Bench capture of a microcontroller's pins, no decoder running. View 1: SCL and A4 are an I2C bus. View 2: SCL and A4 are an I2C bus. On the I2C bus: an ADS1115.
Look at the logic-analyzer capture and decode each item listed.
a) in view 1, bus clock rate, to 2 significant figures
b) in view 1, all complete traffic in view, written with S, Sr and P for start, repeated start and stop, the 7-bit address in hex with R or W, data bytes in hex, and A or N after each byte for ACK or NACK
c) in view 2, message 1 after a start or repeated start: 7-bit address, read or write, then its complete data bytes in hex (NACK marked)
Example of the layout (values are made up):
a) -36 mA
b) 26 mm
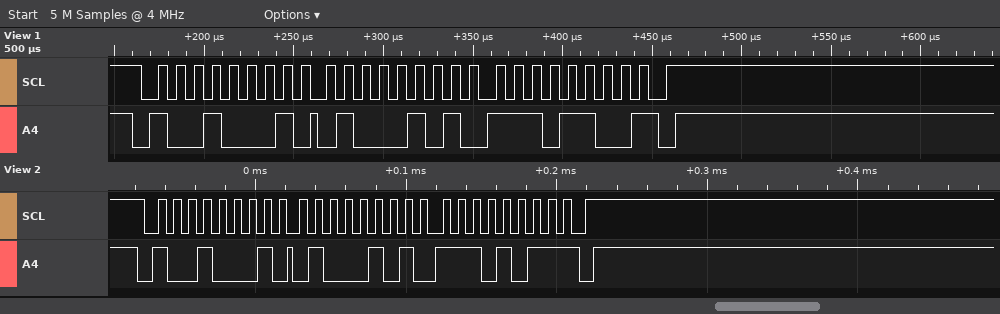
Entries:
a) 100 kHz
b) S 48R A 45 A EC N P
c) 0x48 read: 45 EB NACK
